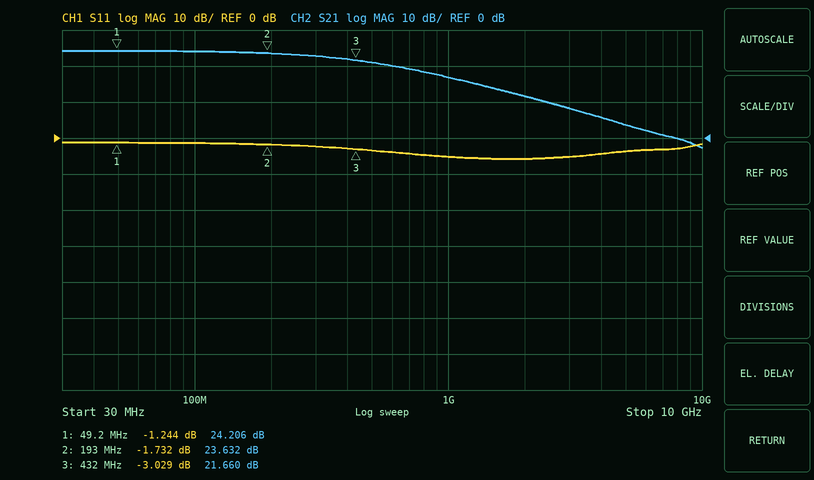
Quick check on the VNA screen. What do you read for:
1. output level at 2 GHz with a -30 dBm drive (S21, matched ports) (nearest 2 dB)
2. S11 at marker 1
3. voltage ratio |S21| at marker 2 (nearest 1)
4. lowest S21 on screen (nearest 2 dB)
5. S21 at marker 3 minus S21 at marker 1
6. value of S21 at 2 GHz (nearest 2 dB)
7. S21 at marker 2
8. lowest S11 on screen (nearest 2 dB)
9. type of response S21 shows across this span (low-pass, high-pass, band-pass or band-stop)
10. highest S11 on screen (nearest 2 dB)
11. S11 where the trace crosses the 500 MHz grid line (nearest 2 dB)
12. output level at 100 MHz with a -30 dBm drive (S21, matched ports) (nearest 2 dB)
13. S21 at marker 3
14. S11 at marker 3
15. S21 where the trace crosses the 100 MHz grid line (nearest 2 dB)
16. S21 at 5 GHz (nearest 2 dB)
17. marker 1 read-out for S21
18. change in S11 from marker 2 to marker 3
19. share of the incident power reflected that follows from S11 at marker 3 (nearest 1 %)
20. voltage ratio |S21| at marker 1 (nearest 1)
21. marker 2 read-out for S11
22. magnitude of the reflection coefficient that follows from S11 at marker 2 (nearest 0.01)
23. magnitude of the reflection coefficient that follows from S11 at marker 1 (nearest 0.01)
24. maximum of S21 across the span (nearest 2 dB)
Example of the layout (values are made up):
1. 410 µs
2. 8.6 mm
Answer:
1. -18 dBm
2. -1.244 dB
3. 15
4. -2 dB
5. -2.546 dB
6. 12 dB
7. 23.632 dB
8. -6 dB
9. low-pass
10. -2 dB
11. -4 dB
12. -6 dBm
13. 21.660 dB
14. -3.029 dB
15. 24 dB
16. 4 dB
17. 24.206 dB
18. -1.297 dB
19. 50 %
20. 16
21. -1.732 dB
22. 0.82
23. 0.87
24. 24 dB
